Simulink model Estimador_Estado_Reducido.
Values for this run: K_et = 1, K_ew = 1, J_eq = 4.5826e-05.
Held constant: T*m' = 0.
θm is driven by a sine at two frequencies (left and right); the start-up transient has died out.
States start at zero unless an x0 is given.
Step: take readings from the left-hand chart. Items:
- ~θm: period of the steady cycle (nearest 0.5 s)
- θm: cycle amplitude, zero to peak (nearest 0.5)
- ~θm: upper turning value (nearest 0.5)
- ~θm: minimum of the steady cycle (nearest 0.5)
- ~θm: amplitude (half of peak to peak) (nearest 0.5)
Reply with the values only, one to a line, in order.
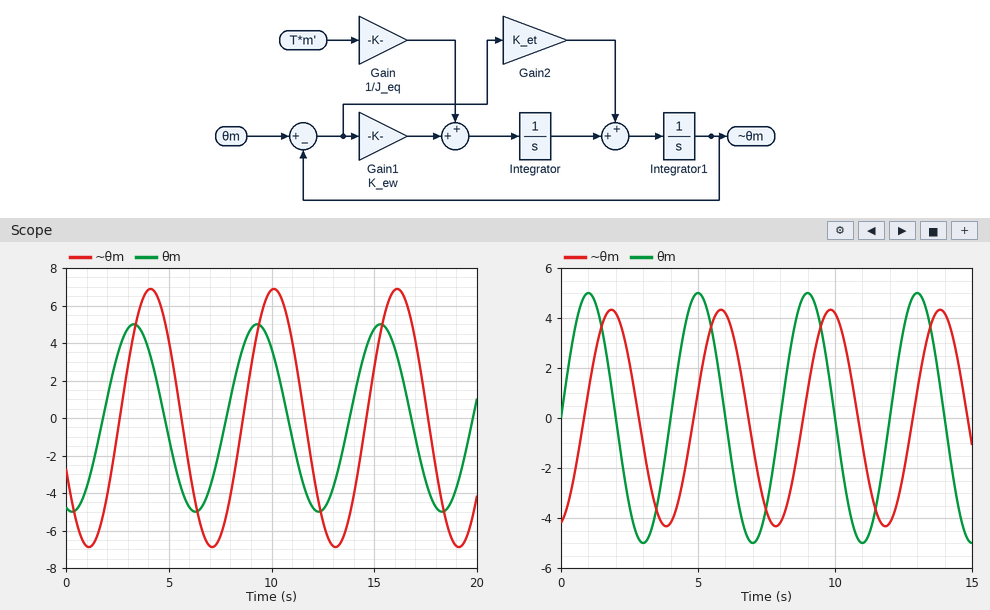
6.0 s
5.0
7.0
-7.0
7.0
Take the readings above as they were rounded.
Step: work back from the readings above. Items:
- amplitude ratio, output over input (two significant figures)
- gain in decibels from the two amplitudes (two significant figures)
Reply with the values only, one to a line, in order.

1.4
2.9 dB
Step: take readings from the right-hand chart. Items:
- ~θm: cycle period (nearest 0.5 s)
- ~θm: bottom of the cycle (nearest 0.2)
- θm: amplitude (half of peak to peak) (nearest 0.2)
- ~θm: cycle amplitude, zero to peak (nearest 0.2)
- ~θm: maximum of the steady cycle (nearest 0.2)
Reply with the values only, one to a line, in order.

4.0 s
-4.4
5.0
4.4
4.4
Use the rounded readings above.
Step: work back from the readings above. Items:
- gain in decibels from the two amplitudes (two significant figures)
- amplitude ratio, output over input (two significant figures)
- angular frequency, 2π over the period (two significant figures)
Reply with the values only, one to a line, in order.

-1.1 dB
0.88
1.6 rad/s
